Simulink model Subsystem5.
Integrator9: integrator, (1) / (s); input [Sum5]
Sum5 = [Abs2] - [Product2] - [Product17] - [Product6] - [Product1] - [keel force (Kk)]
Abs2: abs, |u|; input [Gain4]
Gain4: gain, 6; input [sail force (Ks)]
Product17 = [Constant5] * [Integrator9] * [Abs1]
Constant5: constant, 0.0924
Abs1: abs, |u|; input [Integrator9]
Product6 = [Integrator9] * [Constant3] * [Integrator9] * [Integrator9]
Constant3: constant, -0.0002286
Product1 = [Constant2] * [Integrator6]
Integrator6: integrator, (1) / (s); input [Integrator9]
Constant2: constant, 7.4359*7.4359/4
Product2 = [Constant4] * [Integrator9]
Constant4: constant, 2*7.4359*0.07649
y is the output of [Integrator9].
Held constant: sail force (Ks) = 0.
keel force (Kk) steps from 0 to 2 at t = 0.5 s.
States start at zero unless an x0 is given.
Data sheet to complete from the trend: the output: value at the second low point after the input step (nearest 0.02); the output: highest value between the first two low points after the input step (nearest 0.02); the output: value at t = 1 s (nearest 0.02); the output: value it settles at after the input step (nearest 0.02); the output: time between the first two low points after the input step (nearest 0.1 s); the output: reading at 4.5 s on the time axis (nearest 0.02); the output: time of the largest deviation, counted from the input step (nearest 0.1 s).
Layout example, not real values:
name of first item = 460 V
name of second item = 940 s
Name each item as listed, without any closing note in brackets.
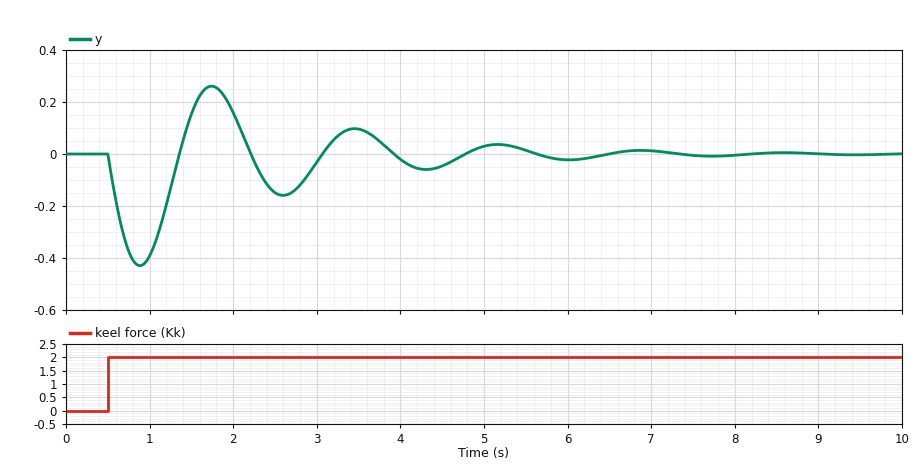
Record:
the output: value at the second low point after the input step = -0.16
the output: highest value between the first two low points after the input step = 0.26
the output: value at t = 1 s = -0.40
the output: value it settles at after the input step = 0.00
the output: time between the first two low points after the input step = 1.7 s
the output: reading at 4.5 s on the time axis = -0.04
the output: time of the largest deviation, counted from the input step = 0.4 s
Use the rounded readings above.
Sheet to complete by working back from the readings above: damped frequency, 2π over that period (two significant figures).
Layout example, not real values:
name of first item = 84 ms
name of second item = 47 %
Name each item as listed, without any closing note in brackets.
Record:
damped frequency, 2π over that period = 3.7 rad/s
